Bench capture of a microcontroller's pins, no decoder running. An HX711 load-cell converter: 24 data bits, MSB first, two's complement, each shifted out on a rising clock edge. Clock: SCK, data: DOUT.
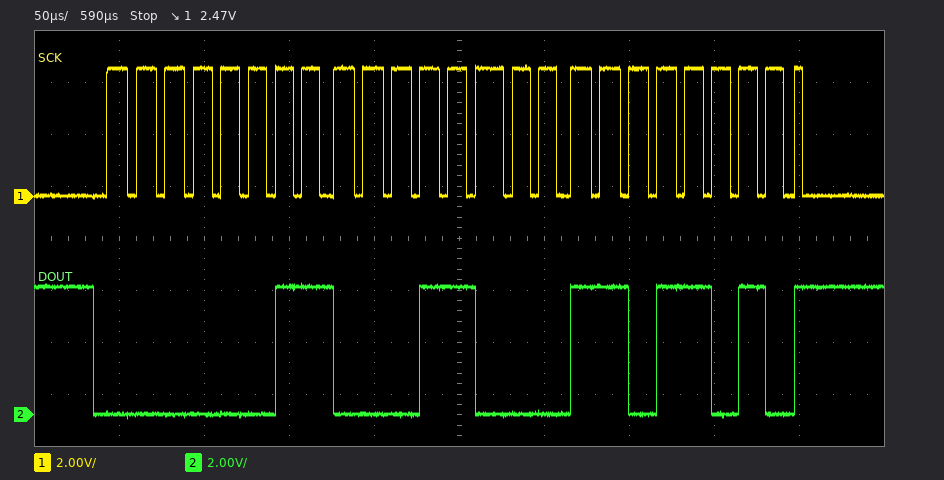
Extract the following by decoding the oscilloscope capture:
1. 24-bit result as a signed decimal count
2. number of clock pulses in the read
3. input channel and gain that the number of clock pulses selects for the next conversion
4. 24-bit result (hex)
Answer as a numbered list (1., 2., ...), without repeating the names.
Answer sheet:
1. 202970
2. 25
3. channel A, gain 128
4. 0x0318DA
